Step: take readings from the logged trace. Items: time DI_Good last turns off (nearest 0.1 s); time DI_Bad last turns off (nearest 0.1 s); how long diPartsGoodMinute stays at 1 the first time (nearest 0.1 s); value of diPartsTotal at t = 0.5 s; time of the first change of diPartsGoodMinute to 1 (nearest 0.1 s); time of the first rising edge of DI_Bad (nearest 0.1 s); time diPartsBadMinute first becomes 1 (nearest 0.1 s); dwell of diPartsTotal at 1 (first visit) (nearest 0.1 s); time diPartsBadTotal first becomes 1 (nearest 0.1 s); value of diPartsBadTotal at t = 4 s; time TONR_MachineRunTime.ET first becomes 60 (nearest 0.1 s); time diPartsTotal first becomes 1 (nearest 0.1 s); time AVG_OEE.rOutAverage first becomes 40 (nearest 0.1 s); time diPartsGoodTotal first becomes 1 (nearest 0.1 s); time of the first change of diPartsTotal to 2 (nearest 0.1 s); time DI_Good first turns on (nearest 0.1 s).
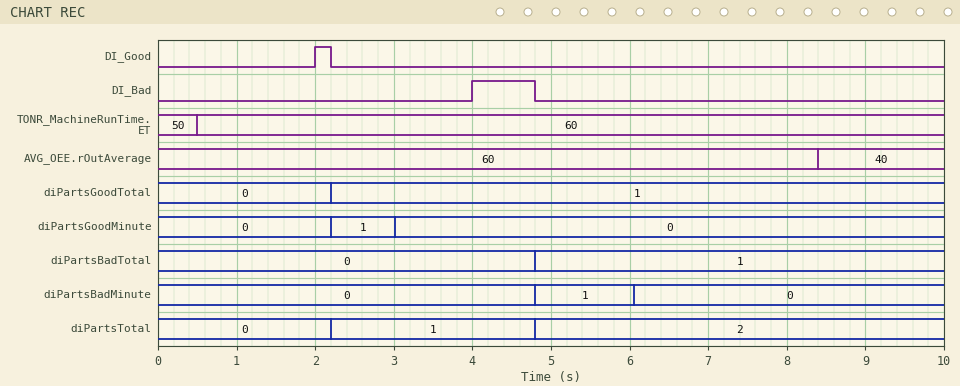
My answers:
2.2 s
4.8 s
0.8 s
0
2.2 s
4.0 s
4.8 s
2.6 s
4.8 s
0
0.5 s
2.2 s
8.4 s
2.2 s
4.8 s
2.0 s
